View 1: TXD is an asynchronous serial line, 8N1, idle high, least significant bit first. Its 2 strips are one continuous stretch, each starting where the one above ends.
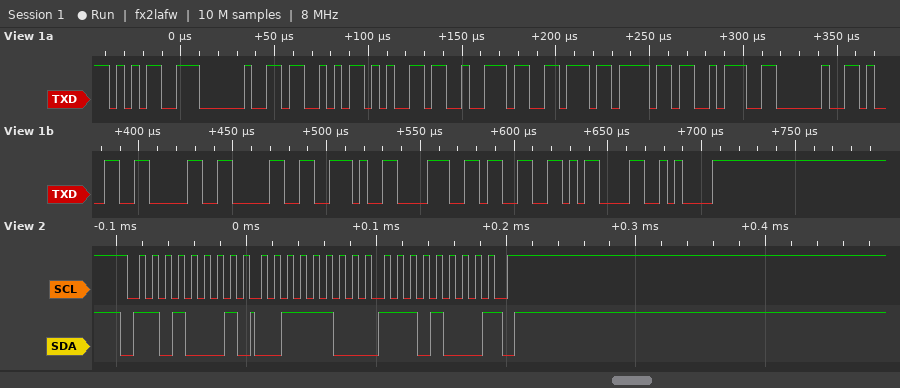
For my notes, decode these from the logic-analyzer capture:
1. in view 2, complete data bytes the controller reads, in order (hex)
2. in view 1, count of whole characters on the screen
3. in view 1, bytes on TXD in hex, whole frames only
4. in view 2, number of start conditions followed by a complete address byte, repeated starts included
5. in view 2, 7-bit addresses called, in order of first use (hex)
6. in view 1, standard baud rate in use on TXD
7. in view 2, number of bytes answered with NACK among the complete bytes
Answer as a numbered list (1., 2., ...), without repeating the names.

1. 3C E8
2. 17
3. 35 20 53 65 72 76 6F 3A 20 31 30 30 2E 38 33 0D 0A
4. 1
5. 0x68
6. 250000 baud
7. 1
